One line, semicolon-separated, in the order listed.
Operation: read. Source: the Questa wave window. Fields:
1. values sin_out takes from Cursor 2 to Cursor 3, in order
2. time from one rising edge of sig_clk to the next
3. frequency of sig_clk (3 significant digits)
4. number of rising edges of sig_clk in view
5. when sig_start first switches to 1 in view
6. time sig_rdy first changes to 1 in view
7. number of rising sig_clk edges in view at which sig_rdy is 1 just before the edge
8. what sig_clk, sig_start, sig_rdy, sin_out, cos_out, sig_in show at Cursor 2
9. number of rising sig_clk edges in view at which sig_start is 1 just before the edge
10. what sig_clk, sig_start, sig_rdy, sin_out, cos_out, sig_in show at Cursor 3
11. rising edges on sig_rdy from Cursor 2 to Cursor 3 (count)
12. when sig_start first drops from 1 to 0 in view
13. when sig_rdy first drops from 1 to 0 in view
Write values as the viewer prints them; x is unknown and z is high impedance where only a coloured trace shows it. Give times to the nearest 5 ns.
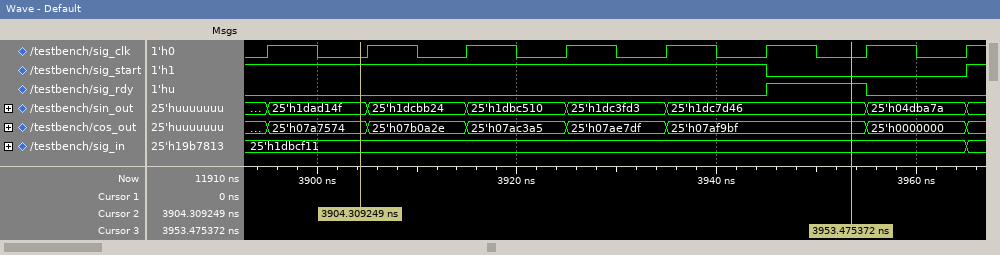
25'h1dad14f, 25'h1dcbb24, 25'h1dbc510, 25'h1dc3fd3, 25'h1dc7d46; 10 ns; 100 MHz; 8; 3965 ns; 3945 ns; 1; sig_clk=0, sig_start=1, sig_rdy=0, sin_out=25'h1dad14f, cos_out=25'h07a7574, sig_in=25'h1dbcf11; 6; sig_clk=0, sig_start=0, sig_rdy=1, sin_out=25'h1dc7d46, cos_out=25'h07af9bf, sig_in=25'h1dbcf11; 1; 3945 ns; 3955 ns
